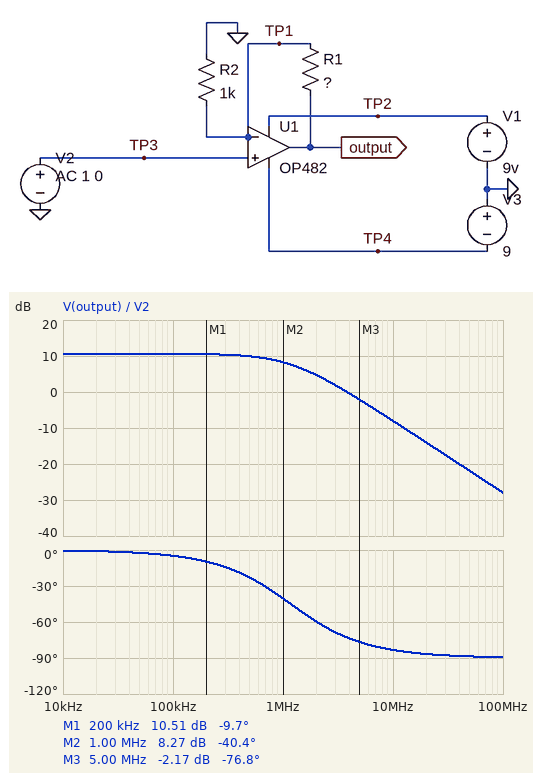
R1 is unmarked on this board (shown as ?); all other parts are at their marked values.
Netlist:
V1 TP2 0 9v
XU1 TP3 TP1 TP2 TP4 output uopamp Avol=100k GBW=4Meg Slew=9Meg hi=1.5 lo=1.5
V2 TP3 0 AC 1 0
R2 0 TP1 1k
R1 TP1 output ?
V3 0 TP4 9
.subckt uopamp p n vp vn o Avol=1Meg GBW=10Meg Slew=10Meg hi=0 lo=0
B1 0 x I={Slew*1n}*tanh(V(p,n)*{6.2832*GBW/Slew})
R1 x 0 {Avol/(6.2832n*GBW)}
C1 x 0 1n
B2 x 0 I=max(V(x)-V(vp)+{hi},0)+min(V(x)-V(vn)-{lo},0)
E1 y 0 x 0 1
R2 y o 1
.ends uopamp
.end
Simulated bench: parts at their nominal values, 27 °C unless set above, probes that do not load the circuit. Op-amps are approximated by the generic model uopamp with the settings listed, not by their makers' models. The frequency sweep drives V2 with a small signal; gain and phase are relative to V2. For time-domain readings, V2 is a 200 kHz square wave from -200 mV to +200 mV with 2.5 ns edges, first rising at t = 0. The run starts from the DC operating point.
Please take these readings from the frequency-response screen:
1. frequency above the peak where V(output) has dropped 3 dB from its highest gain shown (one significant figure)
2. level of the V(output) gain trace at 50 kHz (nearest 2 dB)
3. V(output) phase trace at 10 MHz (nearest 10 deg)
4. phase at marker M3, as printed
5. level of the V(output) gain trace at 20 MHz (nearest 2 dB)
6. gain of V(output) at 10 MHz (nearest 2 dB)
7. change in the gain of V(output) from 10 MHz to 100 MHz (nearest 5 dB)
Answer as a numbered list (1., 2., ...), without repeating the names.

1. 1 MHz
2. 10 dB
3. -80 deg
4. -76.8 deg
5. -14 dB
6. -8 dB
7. -20 dB
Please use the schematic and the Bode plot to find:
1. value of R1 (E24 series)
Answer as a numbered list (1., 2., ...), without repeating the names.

1. 2.4 kΩ
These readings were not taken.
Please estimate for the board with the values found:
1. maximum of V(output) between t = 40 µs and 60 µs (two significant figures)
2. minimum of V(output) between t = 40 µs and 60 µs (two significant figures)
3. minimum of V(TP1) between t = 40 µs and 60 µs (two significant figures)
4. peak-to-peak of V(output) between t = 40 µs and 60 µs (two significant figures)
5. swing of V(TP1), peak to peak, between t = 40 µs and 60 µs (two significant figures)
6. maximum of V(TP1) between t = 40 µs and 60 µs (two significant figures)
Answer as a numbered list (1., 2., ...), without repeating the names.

1. 680 mV
2. -680 mV
3. -200 mV
4. 1.4 V
5. 400 mV
6. 200 mV
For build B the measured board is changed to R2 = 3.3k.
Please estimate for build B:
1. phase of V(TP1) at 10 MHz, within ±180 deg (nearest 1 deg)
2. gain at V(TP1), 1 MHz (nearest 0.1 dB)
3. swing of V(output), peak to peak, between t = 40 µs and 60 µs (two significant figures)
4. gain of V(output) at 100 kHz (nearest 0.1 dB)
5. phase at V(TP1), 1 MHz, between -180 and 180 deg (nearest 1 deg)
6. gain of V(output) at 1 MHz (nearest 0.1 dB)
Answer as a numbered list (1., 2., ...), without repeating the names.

1. -77 deg
2. -0.7 dB
3. 690 mV
4. 4.7 dB
5. -23 deg
6. 4.0 dB
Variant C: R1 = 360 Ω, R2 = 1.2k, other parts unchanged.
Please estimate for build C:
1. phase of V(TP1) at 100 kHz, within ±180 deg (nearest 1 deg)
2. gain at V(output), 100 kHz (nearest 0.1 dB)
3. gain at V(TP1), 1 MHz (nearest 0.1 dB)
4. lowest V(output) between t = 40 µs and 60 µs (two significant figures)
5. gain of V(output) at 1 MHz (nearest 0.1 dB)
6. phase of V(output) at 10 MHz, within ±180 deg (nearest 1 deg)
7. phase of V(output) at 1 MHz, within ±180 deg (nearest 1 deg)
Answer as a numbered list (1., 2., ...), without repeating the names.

1. -2 deg
2. 2.3 dB
3. -0.4 dB
4. -260 mV
5. 1.8 dB
6. -73 deg
7. -18 deg
